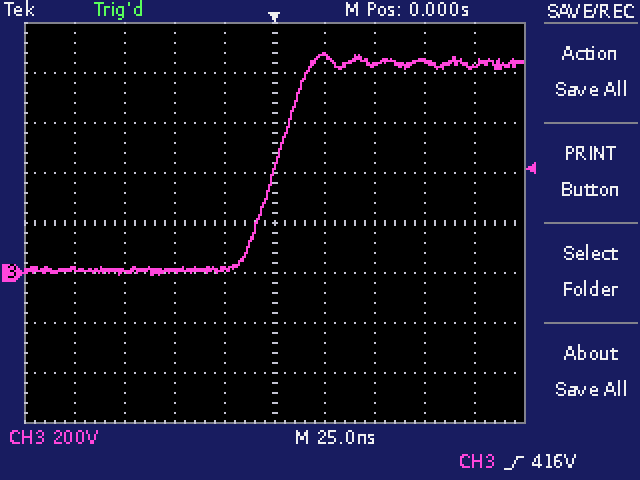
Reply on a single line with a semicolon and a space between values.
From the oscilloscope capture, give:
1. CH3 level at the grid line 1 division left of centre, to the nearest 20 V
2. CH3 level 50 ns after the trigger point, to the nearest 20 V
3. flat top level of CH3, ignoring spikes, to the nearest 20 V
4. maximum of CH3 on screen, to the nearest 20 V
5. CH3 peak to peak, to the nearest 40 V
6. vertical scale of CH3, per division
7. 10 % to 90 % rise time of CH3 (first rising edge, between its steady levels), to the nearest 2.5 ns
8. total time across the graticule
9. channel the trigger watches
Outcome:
20 V; 840 V; 840 V; 880 V; 880 V; 200 V; 27.5 ns; 250 ns; CH3
